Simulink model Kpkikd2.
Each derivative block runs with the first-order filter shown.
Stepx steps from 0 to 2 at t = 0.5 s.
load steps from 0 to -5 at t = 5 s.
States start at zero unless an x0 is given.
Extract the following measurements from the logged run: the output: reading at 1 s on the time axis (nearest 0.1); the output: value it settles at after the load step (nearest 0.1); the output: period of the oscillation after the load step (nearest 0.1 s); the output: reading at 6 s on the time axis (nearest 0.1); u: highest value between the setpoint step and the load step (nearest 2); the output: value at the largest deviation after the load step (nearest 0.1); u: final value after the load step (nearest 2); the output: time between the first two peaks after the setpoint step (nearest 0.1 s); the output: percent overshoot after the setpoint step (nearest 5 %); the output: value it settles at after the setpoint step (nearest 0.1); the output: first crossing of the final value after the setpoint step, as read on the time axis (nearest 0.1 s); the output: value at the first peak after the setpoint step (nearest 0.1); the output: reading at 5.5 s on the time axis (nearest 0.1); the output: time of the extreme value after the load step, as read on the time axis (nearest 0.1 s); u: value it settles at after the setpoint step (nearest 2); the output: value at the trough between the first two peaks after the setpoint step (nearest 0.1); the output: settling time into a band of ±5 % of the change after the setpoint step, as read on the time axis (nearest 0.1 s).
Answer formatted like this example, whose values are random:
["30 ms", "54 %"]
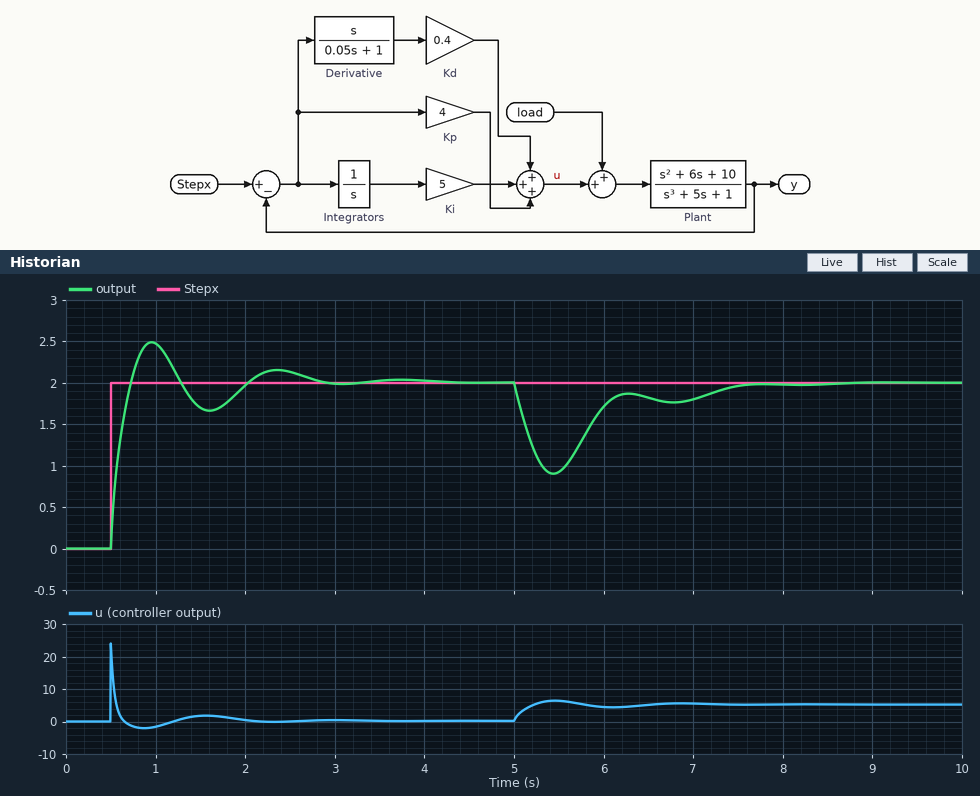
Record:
["2.5", "2.0", "1.3 s", "1.7", "24", "0.9", "6", "1.4 s", "25 %", "2.0", "0.7 s", "2.5", "0.9", "5.4 s", "0", "1.7", "2.6 s"]
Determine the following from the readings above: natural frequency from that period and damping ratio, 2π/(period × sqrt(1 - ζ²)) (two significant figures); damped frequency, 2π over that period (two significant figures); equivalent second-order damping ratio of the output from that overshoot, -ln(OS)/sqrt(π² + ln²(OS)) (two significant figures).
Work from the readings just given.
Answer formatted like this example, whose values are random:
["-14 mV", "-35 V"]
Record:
["4.9 rad/s", "4.5 rad/s", "0.40"]
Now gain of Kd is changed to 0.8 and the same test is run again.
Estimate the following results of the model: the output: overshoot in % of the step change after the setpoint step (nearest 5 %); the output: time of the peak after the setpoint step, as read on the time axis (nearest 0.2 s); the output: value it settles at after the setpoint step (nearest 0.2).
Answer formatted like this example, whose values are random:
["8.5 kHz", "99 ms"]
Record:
["15 %", "1.0 s", "2.0"]
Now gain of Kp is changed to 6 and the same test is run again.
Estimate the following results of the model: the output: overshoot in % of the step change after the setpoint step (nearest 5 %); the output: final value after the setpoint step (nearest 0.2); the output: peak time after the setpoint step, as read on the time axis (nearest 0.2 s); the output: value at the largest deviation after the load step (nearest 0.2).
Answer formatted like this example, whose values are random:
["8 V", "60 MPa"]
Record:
["20 %", "2.0", "0.8 s", "1.2"]
